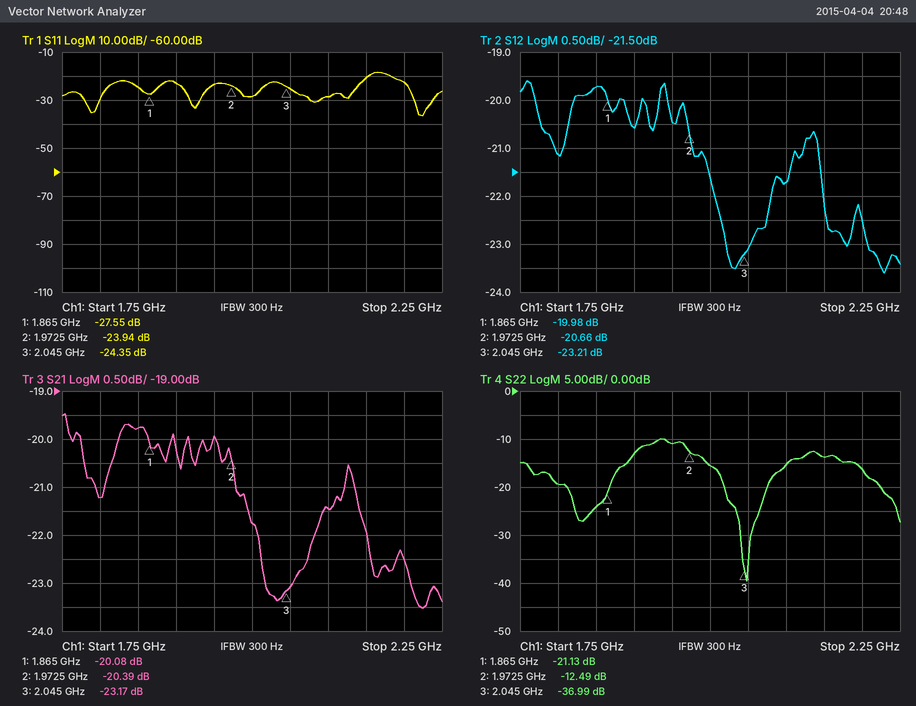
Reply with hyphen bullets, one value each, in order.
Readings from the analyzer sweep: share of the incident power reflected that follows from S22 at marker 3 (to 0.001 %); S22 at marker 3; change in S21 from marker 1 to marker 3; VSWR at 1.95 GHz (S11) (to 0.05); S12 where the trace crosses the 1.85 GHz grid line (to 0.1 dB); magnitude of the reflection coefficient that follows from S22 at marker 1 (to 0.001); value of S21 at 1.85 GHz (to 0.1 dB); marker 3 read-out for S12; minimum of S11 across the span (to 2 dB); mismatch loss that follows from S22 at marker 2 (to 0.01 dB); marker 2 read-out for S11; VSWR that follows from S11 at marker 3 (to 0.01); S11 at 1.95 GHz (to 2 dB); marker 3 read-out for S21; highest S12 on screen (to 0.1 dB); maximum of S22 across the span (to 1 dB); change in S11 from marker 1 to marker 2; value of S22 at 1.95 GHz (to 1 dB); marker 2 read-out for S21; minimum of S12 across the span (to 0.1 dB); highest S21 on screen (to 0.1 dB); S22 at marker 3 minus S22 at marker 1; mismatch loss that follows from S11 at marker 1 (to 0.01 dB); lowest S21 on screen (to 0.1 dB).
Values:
- 0.020 %
- -36.99 dB
- -3.09 dB
- 1.15
- -19.7 dB
- 0.088
- -19.8 dB
- -23.21 dB
- -36 dB
- 0.25 dB
- -23.94 dB
- 1.13
- -24 dB
- -23.17 dB
- -19.6 dB
- -10 dB
- 3.61 dB
- -11 dB
- -20.39 dB
- -23.6 dB
- -19.5 dB
- -15.86 dB
- 0.01 dB
- -23.5 dB
